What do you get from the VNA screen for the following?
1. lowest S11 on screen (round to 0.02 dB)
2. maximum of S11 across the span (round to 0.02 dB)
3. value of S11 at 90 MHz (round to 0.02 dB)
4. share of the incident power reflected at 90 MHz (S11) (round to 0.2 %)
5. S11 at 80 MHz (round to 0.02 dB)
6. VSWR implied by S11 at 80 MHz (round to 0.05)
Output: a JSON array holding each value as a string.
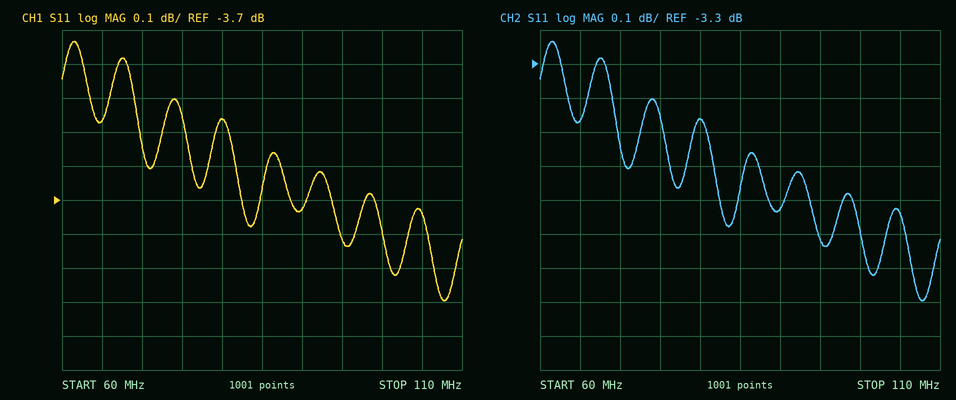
["-4.00 dB", "-3.24 dB", "-3.72 dB", "42.4 %", "-3.46 dB", "5.10"]
